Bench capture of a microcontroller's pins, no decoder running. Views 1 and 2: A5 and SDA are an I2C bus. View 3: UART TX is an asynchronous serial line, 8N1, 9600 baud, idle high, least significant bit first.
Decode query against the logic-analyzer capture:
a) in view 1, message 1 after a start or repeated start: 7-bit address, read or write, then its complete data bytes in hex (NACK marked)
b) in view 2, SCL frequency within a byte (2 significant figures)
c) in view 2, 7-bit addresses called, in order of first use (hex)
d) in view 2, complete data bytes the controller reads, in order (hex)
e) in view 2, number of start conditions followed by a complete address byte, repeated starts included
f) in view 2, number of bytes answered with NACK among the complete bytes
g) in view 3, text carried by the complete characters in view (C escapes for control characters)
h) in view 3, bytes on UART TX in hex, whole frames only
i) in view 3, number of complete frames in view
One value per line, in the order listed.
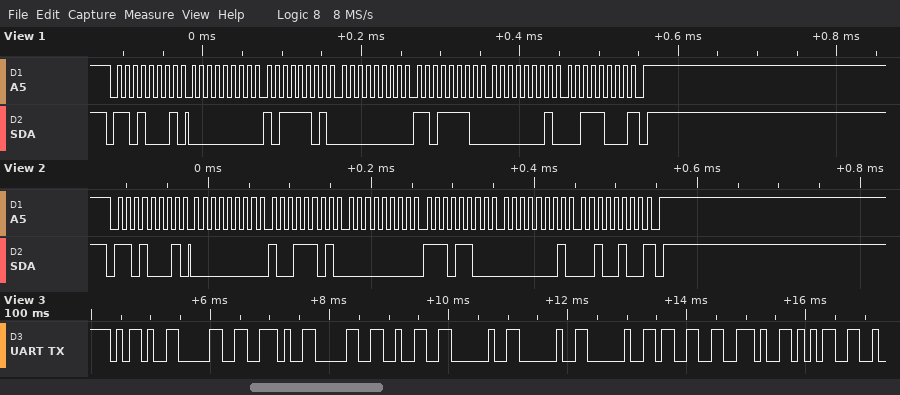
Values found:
0x68 read: 00 BD 00 DE 01 38 NACK
100 kHz
0x68
00 9D 00 EC 01 24
1
1
"-0.02   3.5"
2D 30 2E 30 32 20 20 20 33 2E 35
11
